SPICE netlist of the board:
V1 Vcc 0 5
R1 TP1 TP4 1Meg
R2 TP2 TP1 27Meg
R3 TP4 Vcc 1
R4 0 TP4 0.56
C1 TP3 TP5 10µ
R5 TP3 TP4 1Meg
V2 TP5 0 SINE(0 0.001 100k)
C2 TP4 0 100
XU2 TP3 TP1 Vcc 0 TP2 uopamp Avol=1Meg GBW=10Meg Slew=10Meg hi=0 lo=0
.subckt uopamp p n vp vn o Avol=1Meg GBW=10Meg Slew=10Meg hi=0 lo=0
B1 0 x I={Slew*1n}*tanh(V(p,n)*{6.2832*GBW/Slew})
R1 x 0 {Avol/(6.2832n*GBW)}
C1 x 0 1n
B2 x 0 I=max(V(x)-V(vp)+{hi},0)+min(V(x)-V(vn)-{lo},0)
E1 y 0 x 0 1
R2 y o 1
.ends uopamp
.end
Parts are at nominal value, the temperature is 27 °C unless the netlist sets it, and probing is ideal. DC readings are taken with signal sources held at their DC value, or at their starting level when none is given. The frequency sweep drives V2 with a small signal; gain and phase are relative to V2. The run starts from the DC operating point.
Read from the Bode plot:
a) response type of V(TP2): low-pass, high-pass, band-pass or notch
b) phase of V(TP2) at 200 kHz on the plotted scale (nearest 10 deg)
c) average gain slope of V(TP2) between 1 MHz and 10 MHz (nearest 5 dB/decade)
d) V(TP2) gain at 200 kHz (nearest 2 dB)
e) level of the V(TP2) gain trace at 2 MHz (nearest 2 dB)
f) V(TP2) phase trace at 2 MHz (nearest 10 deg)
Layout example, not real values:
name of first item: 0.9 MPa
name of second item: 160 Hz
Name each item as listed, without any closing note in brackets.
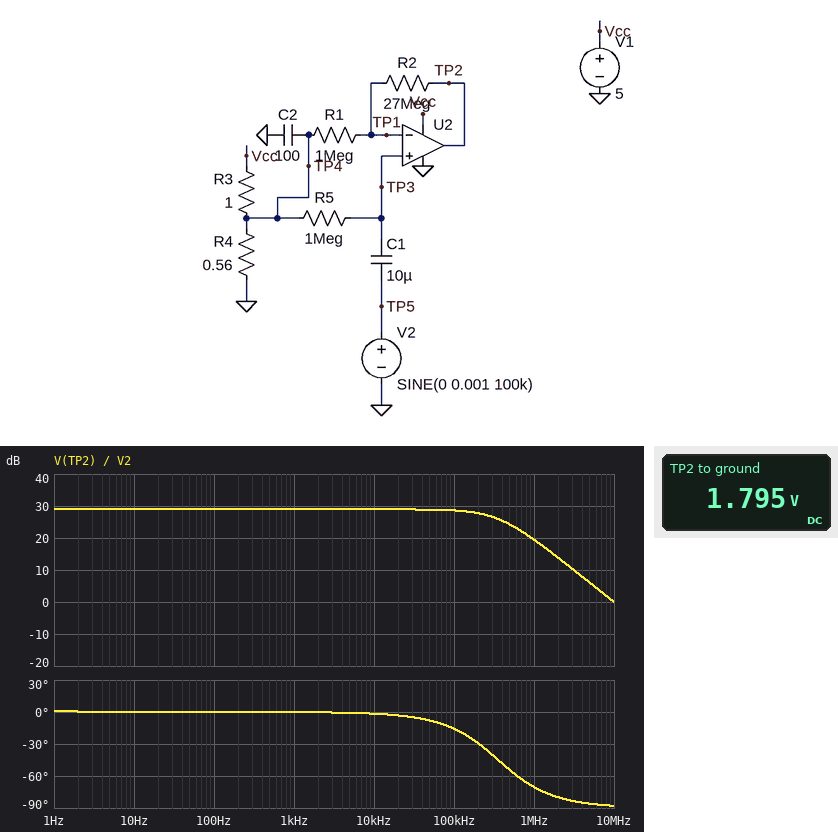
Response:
response type of V(TP2): low-pass, high-pass, band-pass or notch: low-pass
phase of V(TP2) at 200 kHz on the plotted scale: -30 deg
average gain slope of V(TP2) between 1 MHz and 10 MHz: -20 dB/decade
V(TP2) gain at 200 kHz: 28 dB
level of the V(TP2) gain trace at 2 MHz: 14 dB
V(TP2) phase trace at 2 MHz: -80 deg
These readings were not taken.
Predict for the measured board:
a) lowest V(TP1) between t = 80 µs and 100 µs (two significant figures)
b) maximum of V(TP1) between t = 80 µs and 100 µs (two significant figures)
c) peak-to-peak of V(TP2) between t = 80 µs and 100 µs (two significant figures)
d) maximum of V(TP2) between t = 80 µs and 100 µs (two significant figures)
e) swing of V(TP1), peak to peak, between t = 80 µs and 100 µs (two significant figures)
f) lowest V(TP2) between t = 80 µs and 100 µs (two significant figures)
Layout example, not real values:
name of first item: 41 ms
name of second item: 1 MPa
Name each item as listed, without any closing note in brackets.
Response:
lowest V(TP1) between t = 80 µs and 100 µs: 1.8 V
maximum of V(TP1) between t = 80 µs and 100 µs: 1.8 V
peak-to-peak of V(TP2) between t = 80 µs and 100 µs: 54 mV
maximum of V(TP2) between t = 80 µs and 100 µs: 1.8 V
swing of V(TP1), peak to peak, between t = 80 µs and 100 µs: 1.9 mV
lowest V(TP2) between t = 80 µs and 100 µs: 1.8 V
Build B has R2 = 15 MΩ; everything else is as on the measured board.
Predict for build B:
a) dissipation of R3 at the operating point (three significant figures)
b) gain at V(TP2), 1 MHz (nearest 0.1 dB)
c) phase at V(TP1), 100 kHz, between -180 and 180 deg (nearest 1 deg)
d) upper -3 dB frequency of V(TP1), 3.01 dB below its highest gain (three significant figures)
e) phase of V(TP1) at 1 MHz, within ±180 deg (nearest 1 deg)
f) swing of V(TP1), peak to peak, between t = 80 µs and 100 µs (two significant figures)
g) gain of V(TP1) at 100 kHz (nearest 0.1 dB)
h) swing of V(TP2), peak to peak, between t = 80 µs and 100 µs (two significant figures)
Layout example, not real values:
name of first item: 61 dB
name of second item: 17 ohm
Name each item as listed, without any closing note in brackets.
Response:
dissipation of R3 at the operating point: 10.3 W
gain at V(TP2), 1 MHz: 18.6 dB
phase at V(TP1), 100 kHz, between -180 and 180 deg: -9 deg
upper -3 dB frequency of V(TP1), 3.01 dB below its highest gain: 625 kHz
phase of V(TP1) at 1 MHz, within ±180 deg: -58 deg
swing of V(TP1), peak to peak, between t = 80 µs and 100 µs: 2.0 mV
gain of V(TP1) at 100 kHz: -0.1 dB
swing of V(TP2), peak to peak, between t = 80 µs and 100 µs: 32 mV
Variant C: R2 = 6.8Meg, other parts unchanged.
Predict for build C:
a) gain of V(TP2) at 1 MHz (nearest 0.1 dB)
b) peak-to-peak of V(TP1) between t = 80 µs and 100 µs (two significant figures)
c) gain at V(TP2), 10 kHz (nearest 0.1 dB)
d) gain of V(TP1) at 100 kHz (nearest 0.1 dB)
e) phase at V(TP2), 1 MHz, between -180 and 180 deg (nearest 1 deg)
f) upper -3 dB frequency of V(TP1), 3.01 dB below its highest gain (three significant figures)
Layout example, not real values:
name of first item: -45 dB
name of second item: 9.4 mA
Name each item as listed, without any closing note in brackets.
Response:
gain of V(TP2) at 1 MHz: 15.8 dB
peak-to-peak of V(TP1) between t = 80 µs and 100 µs: 2.0 mV
gain at V(TP2), 10 kHz: 17.8 dB
gain of V(TP1) at 100 kHz: 0 dB
phase at V(TP2), 1 MHz, between -180 and 180 deg: -38 deg
upper -3 dB frequency of V(TP1), 3.01 dB below its highest gain: 1.28 MHz
